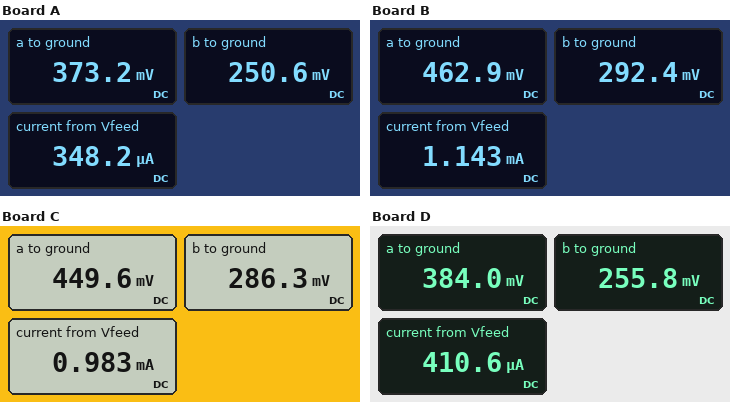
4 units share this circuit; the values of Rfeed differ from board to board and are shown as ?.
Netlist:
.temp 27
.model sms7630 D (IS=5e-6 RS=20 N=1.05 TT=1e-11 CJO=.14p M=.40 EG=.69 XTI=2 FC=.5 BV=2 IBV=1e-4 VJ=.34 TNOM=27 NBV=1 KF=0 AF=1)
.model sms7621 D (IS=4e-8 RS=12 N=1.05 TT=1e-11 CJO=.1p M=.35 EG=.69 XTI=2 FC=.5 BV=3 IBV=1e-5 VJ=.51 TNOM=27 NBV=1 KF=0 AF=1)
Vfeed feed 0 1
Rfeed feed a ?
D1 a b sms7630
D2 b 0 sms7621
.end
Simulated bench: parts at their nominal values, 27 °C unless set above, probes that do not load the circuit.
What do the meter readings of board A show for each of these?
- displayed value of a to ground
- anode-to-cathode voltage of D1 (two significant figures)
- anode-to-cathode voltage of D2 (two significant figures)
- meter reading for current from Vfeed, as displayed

373.2 mV
120 mV
250 mV
348.2 µA
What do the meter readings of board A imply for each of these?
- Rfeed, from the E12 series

1.8 kΩ
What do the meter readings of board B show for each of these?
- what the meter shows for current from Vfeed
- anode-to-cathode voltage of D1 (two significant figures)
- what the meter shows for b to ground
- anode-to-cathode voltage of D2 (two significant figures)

1.143 mA
170 mV
292.4 mV
290 mV
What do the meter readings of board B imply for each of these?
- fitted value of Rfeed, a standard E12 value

470 Ω
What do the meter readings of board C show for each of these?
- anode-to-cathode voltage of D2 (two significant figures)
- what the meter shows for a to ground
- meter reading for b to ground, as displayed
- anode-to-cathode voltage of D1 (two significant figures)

290 mV
449.6 mV
286.3 mV
160 mV
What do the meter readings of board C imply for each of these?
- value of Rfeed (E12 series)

560 Ω
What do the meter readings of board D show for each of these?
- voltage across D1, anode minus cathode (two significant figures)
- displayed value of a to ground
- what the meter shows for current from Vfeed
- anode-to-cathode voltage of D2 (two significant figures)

130 mV
384.0 mV
410.6 µA
260 mV
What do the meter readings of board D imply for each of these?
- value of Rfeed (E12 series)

1.5 kΩ
